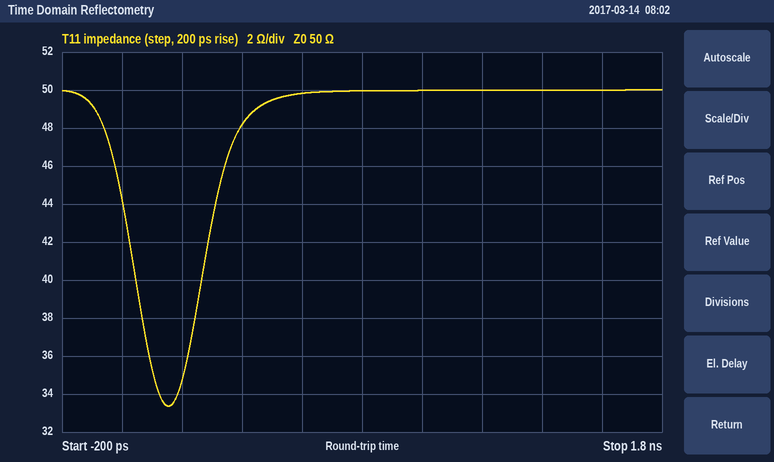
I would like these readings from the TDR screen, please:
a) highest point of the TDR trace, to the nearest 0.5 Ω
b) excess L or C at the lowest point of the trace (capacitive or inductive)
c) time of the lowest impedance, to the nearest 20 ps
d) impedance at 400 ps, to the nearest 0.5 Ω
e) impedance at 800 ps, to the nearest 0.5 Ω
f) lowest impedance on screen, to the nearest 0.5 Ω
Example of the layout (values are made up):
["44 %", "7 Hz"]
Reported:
["50.0 Ω", "capacitive", "160 ps", "48.0 Ω", "50.0 Ω", "33.5 Ω"]
